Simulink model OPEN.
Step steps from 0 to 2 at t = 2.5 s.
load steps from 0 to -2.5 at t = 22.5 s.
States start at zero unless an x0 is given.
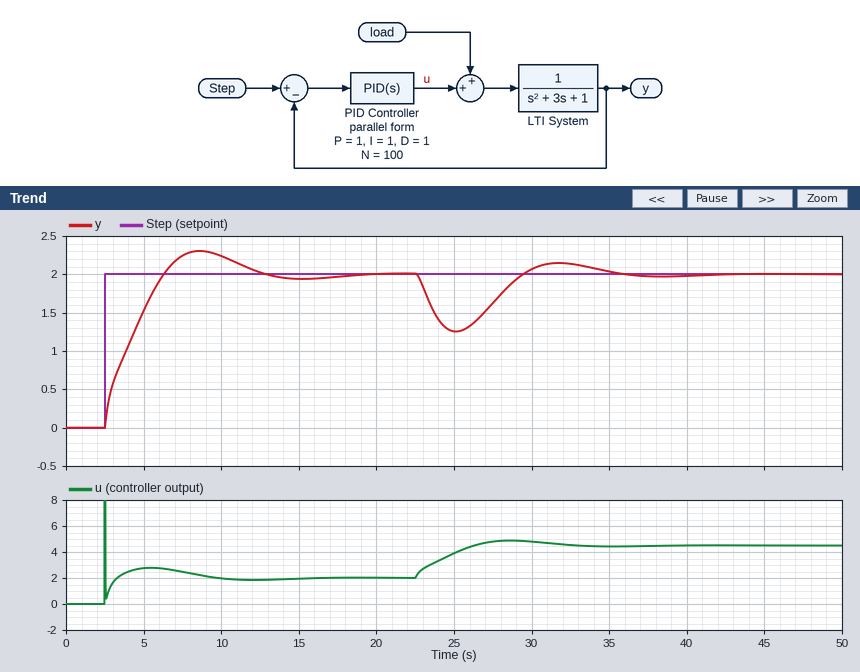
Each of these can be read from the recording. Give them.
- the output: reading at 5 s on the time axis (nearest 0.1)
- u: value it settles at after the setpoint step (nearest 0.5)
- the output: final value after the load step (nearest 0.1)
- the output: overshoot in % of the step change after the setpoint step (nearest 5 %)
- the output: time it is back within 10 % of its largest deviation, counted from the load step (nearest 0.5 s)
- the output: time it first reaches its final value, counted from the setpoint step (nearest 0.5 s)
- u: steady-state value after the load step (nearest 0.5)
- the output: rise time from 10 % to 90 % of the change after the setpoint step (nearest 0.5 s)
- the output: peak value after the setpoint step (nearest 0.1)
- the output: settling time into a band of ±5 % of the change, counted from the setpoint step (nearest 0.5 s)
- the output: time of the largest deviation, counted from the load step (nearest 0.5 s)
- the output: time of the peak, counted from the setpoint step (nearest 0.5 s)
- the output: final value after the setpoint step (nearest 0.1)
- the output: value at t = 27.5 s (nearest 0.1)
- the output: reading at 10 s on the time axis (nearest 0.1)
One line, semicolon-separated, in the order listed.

1.5; 2.0; 2.0; 15 %; 11.5 s; 4.0 s; 4.5; 3.0 s; 2.3; 9.0 s; 2.5 s; 6.0 s; 2.0; 1.6; 2.2
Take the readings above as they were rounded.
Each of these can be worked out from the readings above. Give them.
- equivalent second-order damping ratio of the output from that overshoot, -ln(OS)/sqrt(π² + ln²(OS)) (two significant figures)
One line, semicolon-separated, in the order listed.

0.52
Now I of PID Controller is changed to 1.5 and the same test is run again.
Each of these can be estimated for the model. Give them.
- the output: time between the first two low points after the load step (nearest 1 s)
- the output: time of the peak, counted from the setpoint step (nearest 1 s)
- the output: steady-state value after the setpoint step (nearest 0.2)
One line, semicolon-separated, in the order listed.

10 s; 5 s; 2.0
